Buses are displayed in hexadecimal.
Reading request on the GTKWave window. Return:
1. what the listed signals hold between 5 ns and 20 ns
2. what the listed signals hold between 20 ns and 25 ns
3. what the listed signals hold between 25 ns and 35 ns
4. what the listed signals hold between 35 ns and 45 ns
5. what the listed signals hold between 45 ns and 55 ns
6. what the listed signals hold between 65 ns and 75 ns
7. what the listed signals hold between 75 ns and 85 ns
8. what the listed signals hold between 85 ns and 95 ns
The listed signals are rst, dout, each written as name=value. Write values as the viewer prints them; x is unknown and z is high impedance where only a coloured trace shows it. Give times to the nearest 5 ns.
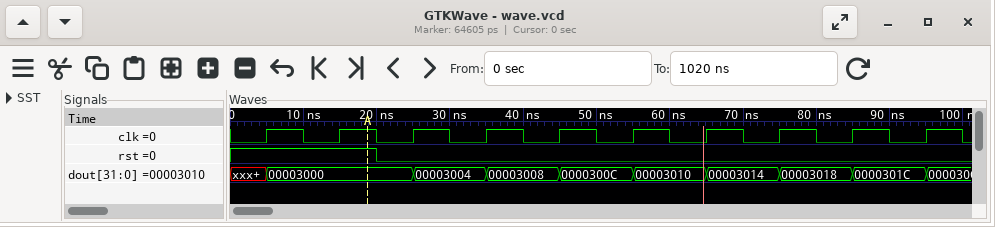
rst=1, dout=00003000
rst=0, dout=00003000
rst=0, dout=00003004
rst=0, dout=00003008
rst=0, dout=0000300C
rst=0, dout=00003014
rst=0, dout=00003018
rst=0, dout=0000301C
